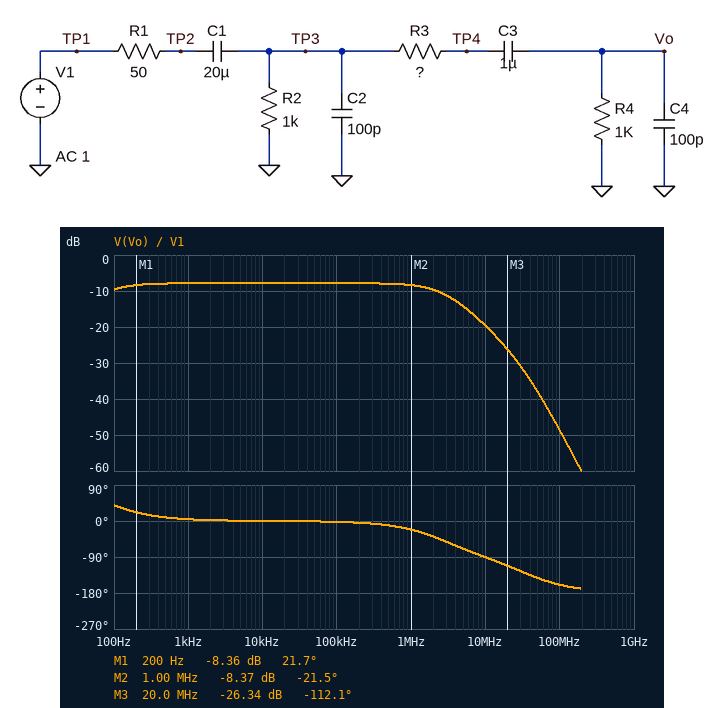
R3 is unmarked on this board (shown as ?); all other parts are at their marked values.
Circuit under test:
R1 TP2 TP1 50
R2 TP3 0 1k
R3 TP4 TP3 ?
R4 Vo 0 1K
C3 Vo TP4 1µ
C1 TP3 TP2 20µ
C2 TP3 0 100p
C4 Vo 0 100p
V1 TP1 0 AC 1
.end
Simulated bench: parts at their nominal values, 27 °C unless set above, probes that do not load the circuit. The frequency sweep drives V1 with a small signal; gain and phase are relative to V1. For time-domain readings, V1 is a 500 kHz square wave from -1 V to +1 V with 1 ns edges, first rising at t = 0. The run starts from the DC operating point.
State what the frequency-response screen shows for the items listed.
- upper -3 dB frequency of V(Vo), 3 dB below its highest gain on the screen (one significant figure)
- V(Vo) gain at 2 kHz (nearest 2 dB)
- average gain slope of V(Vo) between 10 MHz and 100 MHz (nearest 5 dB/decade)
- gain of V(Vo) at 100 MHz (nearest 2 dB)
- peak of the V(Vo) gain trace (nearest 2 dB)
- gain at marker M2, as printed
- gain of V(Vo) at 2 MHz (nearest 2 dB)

3 MHz
-8 dB
-30 dB/decade
-48 dB
-8 dB
-8.37 dB
-10 dB
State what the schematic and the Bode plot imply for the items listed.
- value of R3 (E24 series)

1.3 kΩ
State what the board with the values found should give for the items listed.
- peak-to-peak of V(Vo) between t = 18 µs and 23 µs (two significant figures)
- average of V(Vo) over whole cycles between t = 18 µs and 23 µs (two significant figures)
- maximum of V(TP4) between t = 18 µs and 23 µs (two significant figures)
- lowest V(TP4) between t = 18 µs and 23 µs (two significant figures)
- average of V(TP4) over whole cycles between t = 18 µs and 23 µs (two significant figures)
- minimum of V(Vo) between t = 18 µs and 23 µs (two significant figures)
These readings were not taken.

810 mV
400 mV
820 mV
3.7 mV
410 mV
-4.4 mV
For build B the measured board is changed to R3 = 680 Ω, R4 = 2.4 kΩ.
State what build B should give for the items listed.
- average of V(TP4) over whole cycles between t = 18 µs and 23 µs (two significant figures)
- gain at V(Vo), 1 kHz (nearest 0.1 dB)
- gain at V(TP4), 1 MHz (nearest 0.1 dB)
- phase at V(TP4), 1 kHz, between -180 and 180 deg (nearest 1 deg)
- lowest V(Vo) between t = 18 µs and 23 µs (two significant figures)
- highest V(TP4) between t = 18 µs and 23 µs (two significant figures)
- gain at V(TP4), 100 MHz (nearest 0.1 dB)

730 mV
-2.7 dB
-3.2 dB
0 deg
-6.1 mV
1.5 V
-43.1 dB
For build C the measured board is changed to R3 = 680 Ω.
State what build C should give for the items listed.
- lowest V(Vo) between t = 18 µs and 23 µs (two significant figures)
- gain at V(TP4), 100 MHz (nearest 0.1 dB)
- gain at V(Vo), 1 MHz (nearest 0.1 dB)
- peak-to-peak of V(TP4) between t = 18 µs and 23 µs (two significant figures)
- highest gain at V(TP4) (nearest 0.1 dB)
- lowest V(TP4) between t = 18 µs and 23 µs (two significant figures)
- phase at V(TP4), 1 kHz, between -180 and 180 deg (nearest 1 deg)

-7.9 mV
-43.1 dB
-5.5 dB
1.1 V
-1.3 dB
3.4 mV
-3 deg
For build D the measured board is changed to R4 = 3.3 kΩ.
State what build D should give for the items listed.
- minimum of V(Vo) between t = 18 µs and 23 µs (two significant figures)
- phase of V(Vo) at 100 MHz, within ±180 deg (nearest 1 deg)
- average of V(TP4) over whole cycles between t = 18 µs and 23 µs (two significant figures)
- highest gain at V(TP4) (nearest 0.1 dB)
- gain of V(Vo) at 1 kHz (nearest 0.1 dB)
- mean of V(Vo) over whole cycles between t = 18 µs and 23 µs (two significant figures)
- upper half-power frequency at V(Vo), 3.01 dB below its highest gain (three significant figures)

-4.0 mV
-160 deg
680 mV
-1.9 dB
-3.4 dB
670 mV
1.66 MHz
